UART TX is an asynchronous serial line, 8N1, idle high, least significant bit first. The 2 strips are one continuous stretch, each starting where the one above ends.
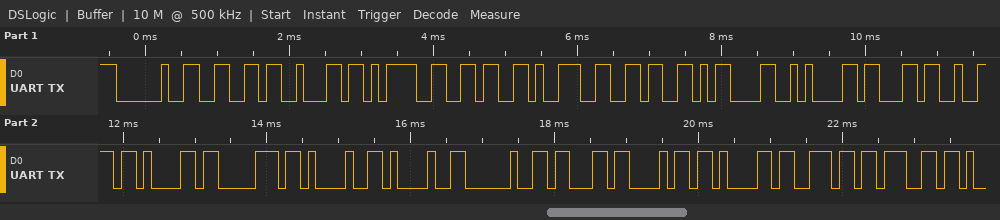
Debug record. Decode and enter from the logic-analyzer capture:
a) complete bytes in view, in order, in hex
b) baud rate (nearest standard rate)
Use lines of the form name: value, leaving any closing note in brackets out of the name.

complete bytes in view, in order, in hex: 20 66 62 3D 36 39 36 0D 0A 63 72 61 70 21 21 20 63 68 61 6E 67
baud rate: 9600 baud
